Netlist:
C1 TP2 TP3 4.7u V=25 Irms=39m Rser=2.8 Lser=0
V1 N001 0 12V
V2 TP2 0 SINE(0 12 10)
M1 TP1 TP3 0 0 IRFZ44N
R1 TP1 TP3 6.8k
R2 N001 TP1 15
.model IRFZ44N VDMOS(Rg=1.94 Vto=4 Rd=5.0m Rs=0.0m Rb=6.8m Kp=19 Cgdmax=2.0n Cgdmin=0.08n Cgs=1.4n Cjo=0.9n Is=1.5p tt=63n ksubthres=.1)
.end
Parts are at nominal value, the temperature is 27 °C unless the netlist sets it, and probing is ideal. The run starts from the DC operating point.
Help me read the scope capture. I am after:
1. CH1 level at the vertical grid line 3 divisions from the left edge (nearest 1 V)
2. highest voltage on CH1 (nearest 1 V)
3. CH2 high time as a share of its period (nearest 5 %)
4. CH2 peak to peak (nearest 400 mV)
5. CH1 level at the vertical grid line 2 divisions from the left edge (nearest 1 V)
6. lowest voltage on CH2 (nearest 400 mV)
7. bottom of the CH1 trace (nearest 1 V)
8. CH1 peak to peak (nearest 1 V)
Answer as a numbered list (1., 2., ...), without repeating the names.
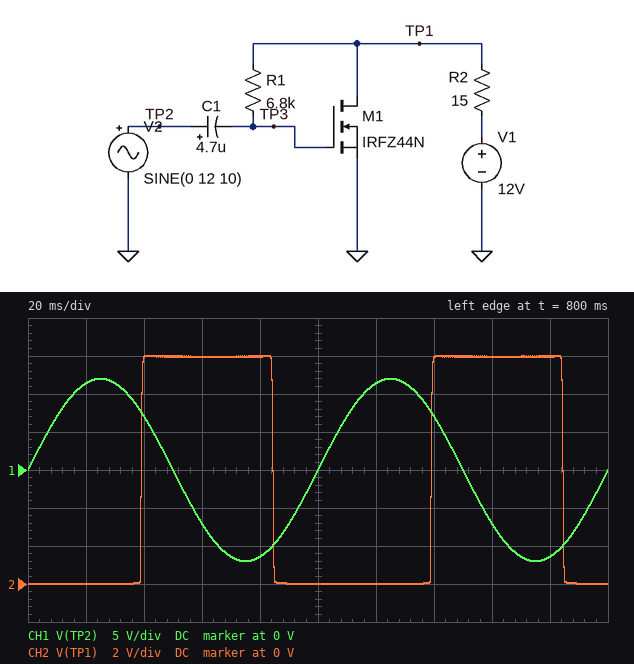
1. -7 V
2. 12 V
3. 45 %
4. 12.0 V
5. 7 V
6. 0 V
7. -12 V
8. 24 V
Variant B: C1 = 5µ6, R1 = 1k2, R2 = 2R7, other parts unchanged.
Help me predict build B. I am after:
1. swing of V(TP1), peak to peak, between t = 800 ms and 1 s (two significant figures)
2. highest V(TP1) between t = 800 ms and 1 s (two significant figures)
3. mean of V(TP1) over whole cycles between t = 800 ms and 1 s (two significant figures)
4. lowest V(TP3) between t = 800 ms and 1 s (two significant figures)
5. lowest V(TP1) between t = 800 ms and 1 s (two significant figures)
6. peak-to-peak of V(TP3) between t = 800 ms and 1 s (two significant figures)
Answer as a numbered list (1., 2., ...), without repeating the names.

1. 9.1 V
2. 9.4 V
3. 4.6 V
4. 4.3 V
5. 240 mV
6. 840 mV
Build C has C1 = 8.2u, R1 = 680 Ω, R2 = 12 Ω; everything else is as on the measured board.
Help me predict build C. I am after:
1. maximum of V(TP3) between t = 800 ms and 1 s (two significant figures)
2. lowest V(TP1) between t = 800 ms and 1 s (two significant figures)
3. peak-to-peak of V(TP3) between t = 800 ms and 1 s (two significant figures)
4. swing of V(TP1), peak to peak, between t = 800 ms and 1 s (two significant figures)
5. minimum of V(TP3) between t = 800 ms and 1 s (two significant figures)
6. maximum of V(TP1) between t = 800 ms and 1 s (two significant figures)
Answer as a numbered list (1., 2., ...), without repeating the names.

1. 4.4 V
2. 190 mV
3. 210 mV
4. 8.2 V
5. 4.2 V
6. 8.4 V
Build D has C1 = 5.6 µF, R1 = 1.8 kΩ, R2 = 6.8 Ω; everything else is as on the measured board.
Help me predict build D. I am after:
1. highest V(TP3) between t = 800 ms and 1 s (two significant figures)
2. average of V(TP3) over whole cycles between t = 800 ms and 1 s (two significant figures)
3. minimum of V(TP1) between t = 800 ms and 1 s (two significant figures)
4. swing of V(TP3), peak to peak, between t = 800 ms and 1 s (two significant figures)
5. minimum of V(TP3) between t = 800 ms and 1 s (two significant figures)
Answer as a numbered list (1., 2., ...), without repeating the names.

1. 6.9 V
2. 4.8 V
3. 41 mV
4. 2.9 V
5. 4.0 V
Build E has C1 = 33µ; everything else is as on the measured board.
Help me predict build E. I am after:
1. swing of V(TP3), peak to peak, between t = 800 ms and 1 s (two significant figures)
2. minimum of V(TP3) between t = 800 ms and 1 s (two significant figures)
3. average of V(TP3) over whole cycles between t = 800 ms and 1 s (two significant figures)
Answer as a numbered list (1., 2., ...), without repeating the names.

1. 24 V
2. -6.4 V
3. 5.5 V
